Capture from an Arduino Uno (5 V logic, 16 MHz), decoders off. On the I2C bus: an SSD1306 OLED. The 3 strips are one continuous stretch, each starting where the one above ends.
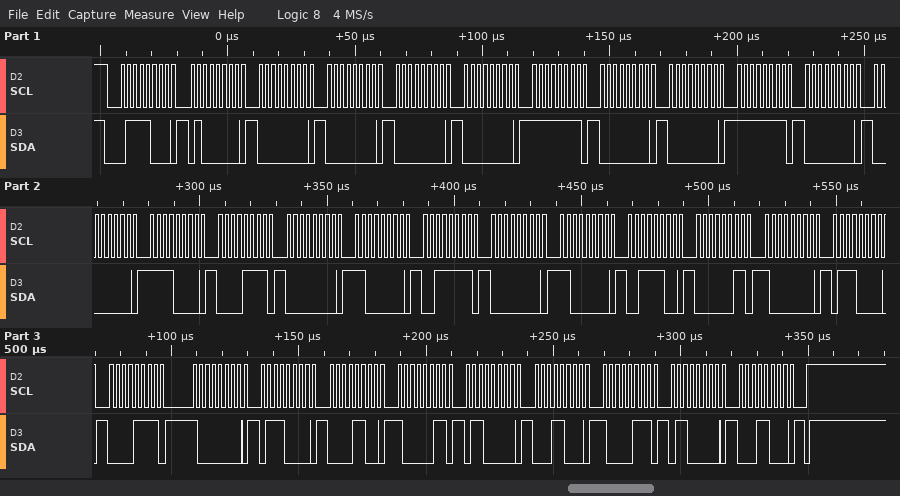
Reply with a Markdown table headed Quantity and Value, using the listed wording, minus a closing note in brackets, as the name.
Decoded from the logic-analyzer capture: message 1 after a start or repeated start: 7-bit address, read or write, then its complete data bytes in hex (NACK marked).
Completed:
| Quantity | Value |
|---|---|
| message 1 after a start or repeated start: 7-bit address, read or write, then its complete data bytes in hex | 0x3C write: 40 00 00 00 00 FF 00 00 FF 00 00 F0 0F 00 C0 3F 00 C0 3C 03 80 70 0F 80 70 0C 83 60 18 87 60 18 |
